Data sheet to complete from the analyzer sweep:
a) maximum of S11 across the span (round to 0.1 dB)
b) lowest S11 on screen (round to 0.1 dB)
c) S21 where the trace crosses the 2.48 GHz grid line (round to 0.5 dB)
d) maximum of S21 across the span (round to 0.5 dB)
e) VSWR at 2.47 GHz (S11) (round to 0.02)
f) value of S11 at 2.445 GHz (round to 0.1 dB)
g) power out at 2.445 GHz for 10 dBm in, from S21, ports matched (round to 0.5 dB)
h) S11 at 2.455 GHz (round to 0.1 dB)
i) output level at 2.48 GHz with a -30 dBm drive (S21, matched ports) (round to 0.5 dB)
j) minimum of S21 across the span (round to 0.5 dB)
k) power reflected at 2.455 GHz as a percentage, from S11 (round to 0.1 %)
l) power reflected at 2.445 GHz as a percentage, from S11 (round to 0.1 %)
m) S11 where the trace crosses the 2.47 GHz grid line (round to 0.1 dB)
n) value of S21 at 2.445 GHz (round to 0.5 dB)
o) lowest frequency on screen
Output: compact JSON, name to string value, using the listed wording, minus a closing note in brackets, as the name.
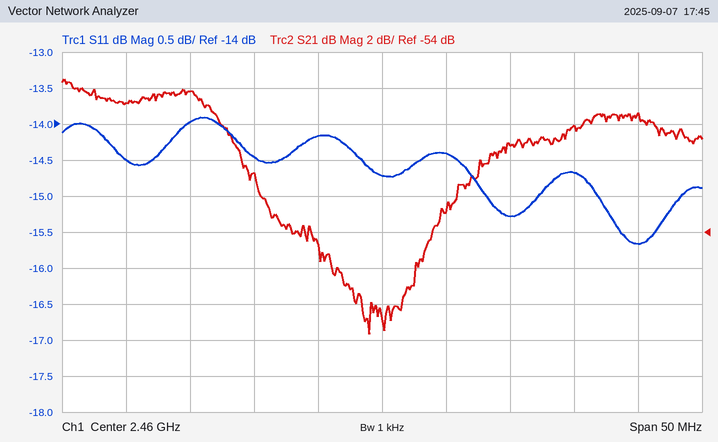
{"maximum of S11 across the span": "-13.9 dB", "lowest S11 on screen": "-15.7 dB", "S21 where the trace crosses the 2.48 GHz grid line": "-47.5 dB", "maximum of S21 across the span": "-45.5 dB", "VSWR at 2.47 GHz (S11)": "1.42", "value of S11 at 2.445 GHz": "-14.0 dB", "power out at 2.445 GHz for 10 dBm in, from S21, ports matched": "-36.0 dBm", "S11 at 2.455 GHz": "-14.2 dB", "output level at 2.48 GHz with a -30 dBm drive (S21, matched ports)": "-77.5 dBm", "minimum of S21 across the span": "-59.5 dB", "power reflected at 2.455 GHz as a percentage, from S11": "3.8 %", "power reflected at 2.445 GHz as a percentage, from S11": "4.0 %", "S11 where the trace crosses the 2.47 GHz grid line": "-15.3 dB", "value of S21 at 2.445 GHz": "-46.0 dB", "lowest frequency on screen": "2.435 GHz"}
